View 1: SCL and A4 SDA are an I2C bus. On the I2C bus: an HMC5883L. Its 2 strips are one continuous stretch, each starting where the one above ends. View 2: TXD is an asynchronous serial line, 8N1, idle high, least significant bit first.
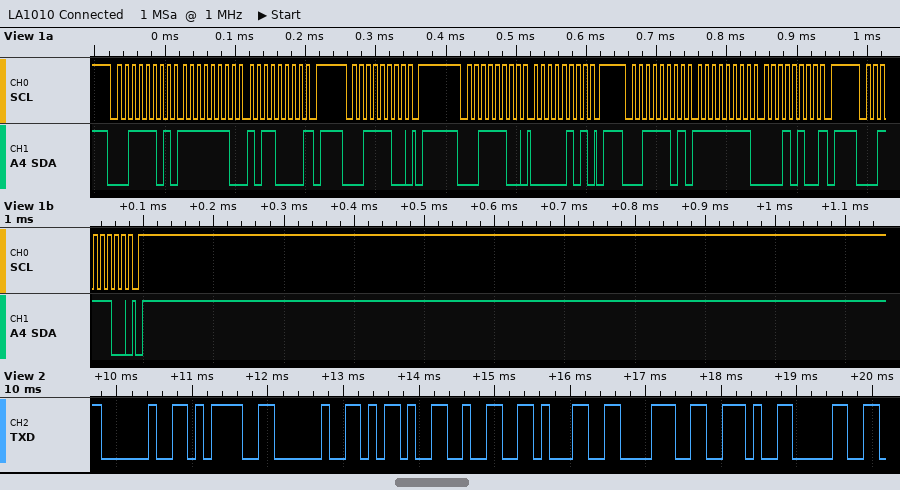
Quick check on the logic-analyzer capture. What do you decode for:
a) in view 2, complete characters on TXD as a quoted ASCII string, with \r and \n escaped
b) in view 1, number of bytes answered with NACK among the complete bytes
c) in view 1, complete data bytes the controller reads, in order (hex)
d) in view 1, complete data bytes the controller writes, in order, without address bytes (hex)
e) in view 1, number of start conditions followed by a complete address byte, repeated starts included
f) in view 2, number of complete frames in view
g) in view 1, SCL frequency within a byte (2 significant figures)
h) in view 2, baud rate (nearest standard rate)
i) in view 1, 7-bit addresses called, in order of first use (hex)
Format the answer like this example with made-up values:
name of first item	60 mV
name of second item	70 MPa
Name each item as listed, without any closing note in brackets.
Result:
in view 2, complete characters on TXD as a quoted ASCII string, with \r and \n escaped	" = -218.0"
in view 1, number of bytes answered with NACK among the complete bytes	2
in view 1, complete data bytes the controller reads, in order	FE B0 FF 14
in view 1, complete data bytes the controller writes, in order, without address bytes	05
in view 1, number of start conditions followed by a complete address byte, repeated starts included	5
in view 2, number of complete frames in view	9
in view 1, SCL frequency within a byte	100 kHz
in view 2, baud rate	9600 baud
in view 1, 7-bit addresses called, in order of first use	0x1E
